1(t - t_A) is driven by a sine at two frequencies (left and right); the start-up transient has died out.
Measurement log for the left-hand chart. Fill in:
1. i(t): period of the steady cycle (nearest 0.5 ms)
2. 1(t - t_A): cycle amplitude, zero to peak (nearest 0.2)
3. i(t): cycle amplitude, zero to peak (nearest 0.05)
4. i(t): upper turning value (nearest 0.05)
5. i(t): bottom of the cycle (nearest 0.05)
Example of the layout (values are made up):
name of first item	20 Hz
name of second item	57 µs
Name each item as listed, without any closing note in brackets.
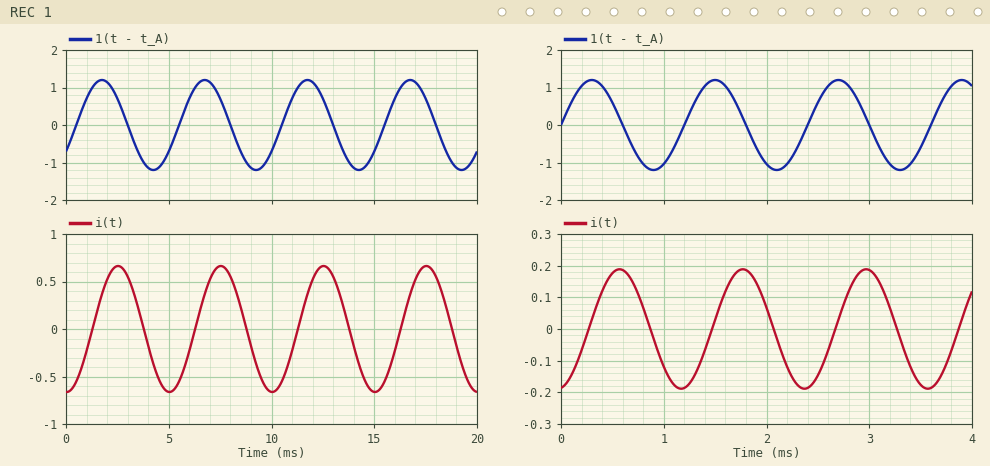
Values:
i(t): period of the steady cycle	5.0 ms
1(t - t_A): cycle amplitude, zero to peak	1.2
i(t): cycle amplitude, zero to peak	0.65
i(t): upper turning value	0.65
i(t): bottom of the cycle	-0.65
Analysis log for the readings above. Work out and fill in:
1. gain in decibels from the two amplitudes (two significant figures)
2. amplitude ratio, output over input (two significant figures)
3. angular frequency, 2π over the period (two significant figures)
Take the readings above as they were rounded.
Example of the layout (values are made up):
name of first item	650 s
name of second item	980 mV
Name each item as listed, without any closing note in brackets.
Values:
gain in decibels from the two amplitudes	-5.3 dB
amplitude ratio, output over input	0.54
angular frequency, 2π over the period	1.3 rad/ms
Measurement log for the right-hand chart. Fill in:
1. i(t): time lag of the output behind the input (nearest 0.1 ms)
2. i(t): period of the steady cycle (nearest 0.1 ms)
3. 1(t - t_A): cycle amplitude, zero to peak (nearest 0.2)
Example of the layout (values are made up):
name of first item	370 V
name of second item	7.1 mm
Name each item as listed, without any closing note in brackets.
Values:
i(t): time lag of the output behind the input	0.3 ms
i(t): period of the steady cycle	1.2 ms
1(t - t_A): cycle amplitude, zero to peak	1.2
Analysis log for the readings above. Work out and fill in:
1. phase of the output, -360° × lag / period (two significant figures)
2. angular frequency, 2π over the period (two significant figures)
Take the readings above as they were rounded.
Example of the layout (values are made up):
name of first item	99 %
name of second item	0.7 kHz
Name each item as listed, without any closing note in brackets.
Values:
phase of the output, -360° × lag / period	-90°
angular frequency, 2π over the period	5.2 rad/ms
